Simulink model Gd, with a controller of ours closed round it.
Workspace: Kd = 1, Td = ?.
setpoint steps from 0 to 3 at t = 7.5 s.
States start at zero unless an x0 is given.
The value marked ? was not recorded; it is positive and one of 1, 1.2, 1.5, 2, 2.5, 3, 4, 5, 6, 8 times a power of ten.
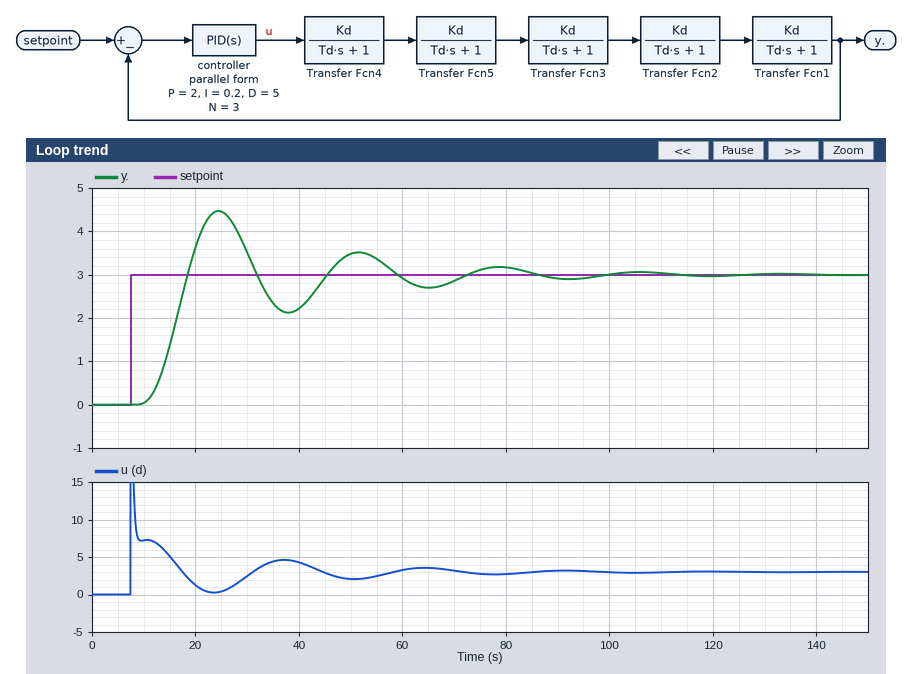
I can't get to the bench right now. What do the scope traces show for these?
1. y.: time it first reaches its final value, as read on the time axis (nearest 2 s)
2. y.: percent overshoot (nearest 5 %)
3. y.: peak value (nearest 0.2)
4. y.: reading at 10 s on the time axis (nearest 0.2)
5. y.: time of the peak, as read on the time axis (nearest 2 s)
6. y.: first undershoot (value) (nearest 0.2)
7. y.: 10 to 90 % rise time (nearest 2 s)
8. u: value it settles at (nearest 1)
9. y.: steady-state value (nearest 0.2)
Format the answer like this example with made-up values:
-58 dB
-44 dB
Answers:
18 s
50 %
4.4
0.0
24 s
2.2
6 s
3
3.0
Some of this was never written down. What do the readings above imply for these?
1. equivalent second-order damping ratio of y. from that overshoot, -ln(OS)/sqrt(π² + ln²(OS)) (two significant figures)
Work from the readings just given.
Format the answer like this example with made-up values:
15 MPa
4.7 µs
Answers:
0.22
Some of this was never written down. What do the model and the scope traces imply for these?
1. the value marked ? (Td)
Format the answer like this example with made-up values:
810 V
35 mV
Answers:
3
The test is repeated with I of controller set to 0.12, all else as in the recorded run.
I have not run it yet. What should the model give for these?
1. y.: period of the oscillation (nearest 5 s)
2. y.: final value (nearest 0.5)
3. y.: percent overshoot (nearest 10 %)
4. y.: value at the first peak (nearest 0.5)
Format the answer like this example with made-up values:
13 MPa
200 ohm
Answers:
25 s
3.0
30 %
4.0
